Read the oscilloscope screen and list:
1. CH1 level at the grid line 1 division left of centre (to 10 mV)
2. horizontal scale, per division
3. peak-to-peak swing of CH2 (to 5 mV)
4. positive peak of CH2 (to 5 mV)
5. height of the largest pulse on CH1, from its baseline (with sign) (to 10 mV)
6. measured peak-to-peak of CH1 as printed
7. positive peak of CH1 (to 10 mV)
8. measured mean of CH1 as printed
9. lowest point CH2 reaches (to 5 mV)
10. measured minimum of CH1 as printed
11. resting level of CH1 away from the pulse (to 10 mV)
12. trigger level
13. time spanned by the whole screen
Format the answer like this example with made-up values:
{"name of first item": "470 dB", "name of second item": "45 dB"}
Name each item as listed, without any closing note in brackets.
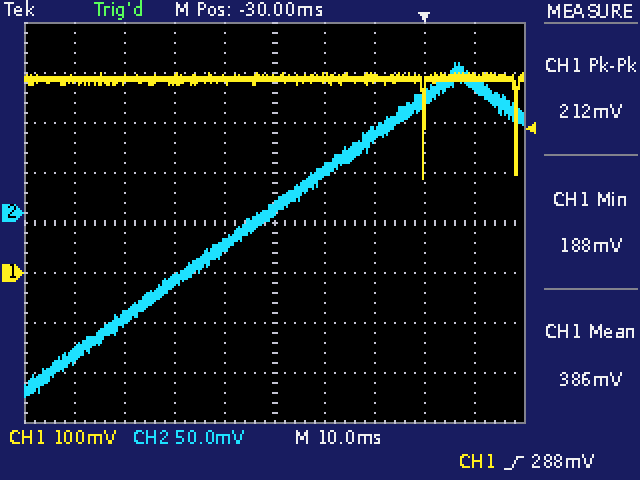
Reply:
{"CH1 level at the grid line 1 division left of centre": "390 mV", "horizontal scale, per division": "10 ms", "peak-to-peak swing of CH2": "335 mV", "positive peak of CH2": "150 mV", "height of the largest pulse on CH1, from its baseline (with sign)": "-200 mV", "measured peak-to-peak of CH1 as printed": "212 mV", "positive peak of CH1": "400 mV", "measured mean of CH1 as printed": "386 mV", "lowest point CH2 reaches": "-185 mV", "measured minimum of CH1 as printed": "188 mV", "resting level of CH1 away from the pulse": "390 mV", "trigger level": "288 mV", "time spanned by the whole screen": "100 ms"}
